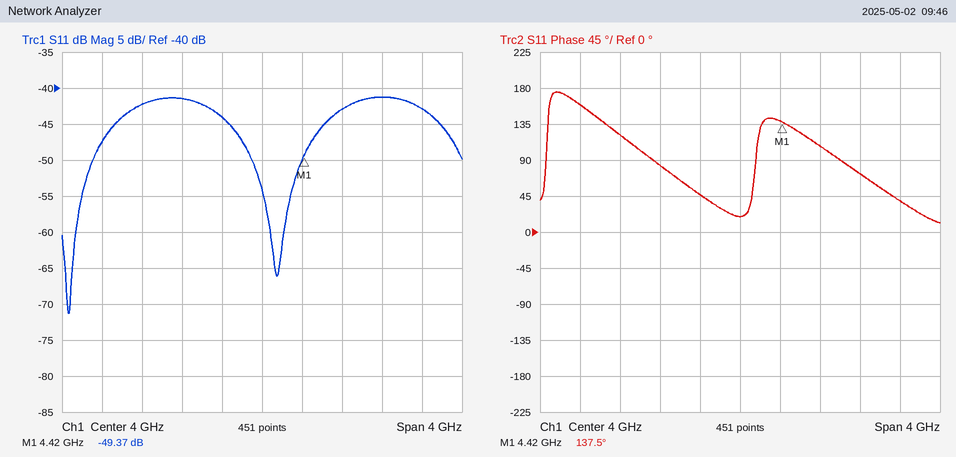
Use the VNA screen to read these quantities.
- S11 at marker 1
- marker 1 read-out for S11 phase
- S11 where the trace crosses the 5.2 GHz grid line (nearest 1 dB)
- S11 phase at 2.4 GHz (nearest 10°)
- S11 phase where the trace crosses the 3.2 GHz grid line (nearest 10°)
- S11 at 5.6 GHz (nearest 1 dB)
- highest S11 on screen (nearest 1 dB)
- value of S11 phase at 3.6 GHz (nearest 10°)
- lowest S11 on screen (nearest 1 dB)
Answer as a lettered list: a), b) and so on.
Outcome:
a) -49.37 dB
b) 137.5°
c) -41 dB
d) 160°
e) 80°
f) -43 dB
g) -41 dB
h) 50°
i) -71 dB
